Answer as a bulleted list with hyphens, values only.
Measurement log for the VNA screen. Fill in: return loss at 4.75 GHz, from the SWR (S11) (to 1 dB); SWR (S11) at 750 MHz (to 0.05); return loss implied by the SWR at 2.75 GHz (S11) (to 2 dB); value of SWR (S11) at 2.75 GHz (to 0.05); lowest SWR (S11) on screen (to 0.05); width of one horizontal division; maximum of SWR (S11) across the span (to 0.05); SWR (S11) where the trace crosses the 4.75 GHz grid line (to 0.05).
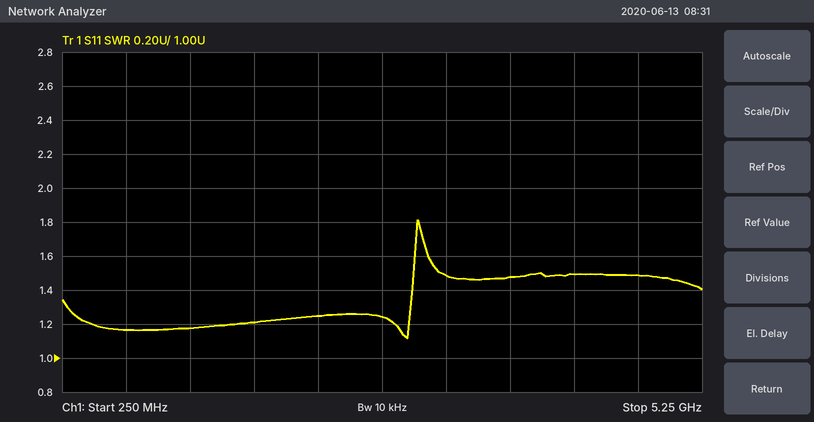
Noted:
- 14 dB
- 1.15
- 20 dB
- 1.25
- 1.10
- 500 MHz
- 1.80
- 1.50
